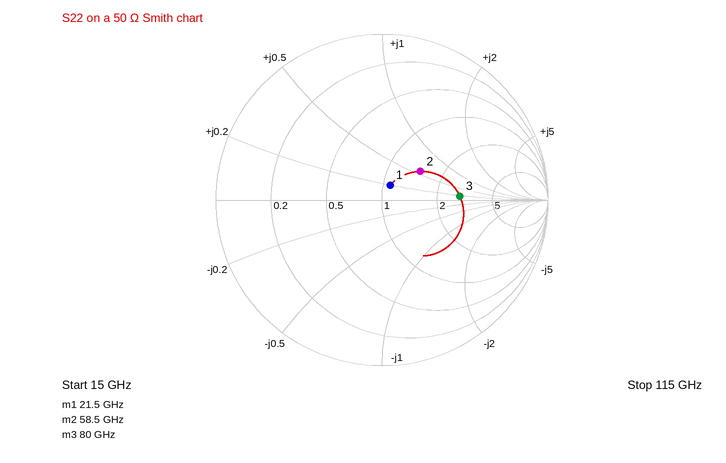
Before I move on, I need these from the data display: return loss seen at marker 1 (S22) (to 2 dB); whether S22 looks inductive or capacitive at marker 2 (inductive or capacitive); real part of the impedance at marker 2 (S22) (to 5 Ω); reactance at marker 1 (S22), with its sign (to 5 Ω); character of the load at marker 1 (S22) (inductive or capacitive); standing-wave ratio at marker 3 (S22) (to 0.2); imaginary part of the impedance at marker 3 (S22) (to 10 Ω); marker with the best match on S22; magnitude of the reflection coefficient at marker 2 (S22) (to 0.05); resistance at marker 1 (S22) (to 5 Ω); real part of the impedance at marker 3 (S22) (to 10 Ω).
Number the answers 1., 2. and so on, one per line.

1. 20 dB
2. inductive
3. 75 Ω
4. +10 Ω
5. inductive
6. 2.8
7. +10 Ω
8. marker 1
9. 0.30
10. 55 Ω
11. 140 Ω
